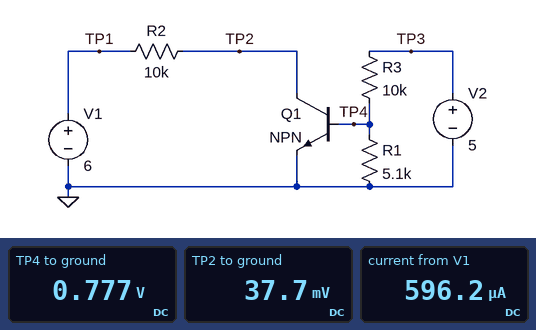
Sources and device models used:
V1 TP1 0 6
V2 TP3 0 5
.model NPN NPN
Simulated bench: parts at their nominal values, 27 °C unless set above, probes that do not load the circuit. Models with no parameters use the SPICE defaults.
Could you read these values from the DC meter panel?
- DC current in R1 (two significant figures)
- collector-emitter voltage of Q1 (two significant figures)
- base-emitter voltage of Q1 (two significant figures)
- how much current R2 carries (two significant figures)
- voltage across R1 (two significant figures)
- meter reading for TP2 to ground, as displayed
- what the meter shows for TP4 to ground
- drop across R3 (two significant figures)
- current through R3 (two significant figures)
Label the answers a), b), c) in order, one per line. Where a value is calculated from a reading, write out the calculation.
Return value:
a) (777 mV) / 5.1 kΩ = 150 µA
b) 37.7 mV = 38 mV
c) 777 mV = 780 mV
d) (6 V - 37.7 mV) / 10 kΩ = 600 µA
e) 777 mV = 780 mV
f) 37.7 mV
g) 0.777 V
h) 5 V - 777 mV = 4.2 V
i) (5 V - 777 mV) / 10 kΩ = 420 µA
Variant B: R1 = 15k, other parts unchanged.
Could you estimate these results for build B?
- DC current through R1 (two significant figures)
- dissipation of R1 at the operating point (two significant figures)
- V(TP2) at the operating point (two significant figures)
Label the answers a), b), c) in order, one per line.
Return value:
a) 52 µA
b) 41 µW
c) 34 mV
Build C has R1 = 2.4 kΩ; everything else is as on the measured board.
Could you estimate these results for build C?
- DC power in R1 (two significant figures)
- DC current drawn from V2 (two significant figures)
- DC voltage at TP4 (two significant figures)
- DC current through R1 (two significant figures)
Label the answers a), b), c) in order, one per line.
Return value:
a) 250 µW
b) 420 µA
c) 770 mV
d) 320 µA
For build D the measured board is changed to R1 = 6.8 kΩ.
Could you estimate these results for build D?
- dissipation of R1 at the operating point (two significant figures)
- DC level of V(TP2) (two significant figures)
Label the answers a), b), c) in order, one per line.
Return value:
a) 89 µW
b) 36 mV
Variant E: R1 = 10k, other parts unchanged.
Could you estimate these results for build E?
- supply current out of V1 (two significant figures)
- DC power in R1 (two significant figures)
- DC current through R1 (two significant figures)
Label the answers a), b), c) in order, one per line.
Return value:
a) 600 µA
b) 61 µW
c) 78 µA
